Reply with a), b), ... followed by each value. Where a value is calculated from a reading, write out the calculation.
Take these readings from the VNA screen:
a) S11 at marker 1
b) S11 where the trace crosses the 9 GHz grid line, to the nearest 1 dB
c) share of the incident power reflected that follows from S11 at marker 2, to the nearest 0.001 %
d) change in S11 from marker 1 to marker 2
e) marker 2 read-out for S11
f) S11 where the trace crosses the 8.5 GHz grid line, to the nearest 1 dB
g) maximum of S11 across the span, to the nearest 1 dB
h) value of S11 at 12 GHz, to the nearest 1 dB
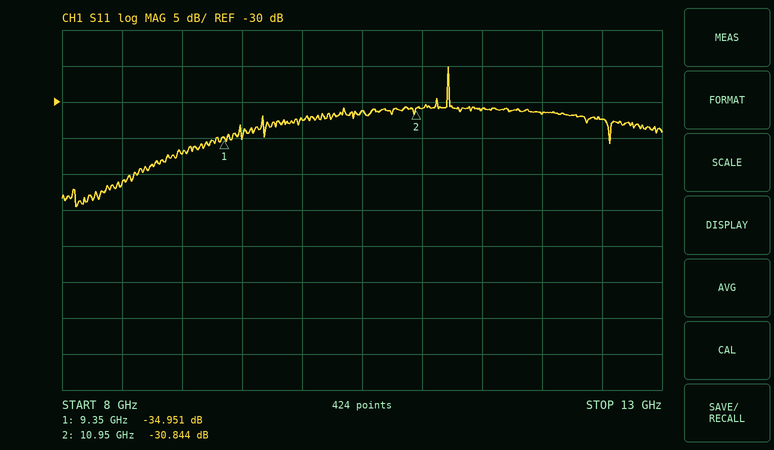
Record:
a) -34.951 dB
b) -37 dB
c) 10^(-30.844/10) ≈ 0.082 %
d) -30.844 − (-34.951) = 4.107 dB
e) -30.844 dB
f) -41 dB
g) -25 dB
h) -32 dB
